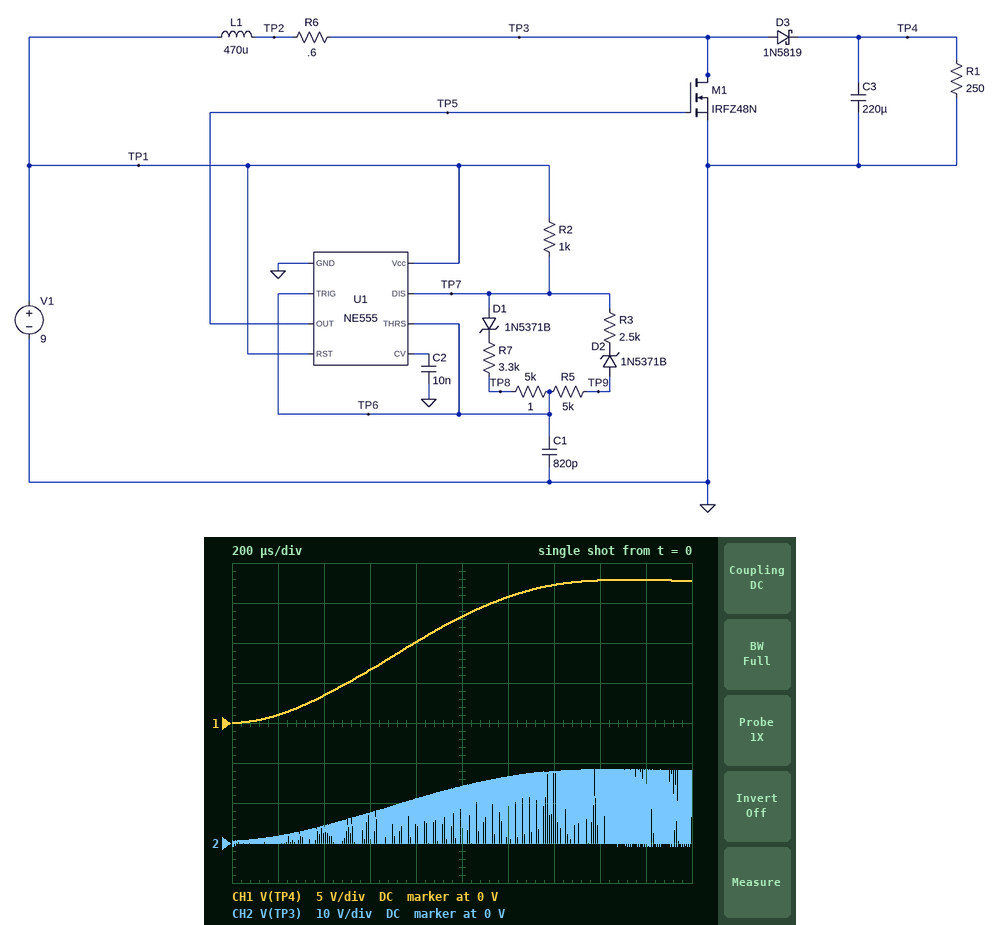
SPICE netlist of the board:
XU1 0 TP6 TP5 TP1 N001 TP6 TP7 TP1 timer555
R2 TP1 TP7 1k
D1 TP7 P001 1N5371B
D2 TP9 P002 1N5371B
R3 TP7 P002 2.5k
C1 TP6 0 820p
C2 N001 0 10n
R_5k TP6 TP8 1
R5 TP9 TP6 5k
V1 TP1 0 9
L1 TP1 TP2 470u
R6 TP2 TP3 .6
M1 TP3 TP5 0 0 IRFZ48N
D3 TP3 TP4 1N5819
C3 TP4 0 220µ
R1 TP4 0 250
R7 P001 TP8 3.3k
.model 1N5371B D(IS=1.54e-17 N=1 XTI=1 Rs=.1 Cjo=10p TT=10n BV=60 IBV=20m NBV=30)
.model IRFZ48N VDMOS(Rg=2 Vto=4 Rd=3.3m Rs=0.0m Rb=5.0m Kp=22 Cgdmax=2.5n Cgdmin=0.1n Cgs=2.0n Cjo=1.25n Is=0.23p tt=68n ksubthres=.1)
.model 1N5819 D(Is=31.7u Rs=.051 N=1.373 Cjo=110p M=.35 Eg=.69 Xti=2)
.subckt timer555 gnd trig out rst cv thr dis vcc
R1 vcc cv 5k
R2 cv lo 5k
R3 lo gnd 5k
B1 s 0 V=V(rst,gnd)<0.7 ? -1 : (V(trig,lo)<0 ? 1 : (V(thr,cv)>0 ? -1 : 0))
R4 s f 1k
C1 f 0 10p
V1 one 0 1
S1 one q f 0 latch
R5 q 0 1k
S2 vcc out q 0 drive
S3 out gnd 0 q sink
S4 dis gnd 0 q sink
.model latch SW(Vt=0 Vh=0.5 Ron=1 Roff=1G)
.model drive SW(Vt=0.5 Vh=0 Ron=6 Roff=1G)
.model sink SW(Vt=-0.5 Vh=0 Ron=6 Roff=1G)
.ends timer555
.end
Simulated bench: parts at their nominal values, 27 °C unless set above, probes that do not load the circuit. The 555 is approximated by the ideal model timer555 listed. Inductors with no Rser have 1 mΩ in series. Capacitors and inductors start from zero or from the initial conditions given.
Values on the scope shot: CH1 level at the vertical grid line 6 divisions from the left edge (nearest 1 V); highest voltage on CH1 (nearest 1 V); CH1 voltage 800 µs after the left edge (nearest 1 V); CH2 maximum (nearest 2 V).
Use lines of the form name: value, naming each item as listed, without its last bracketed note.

CH1 level at the vertical grid line 6 divisions from the left edge: 16 V
highest voltage on CH1: 18 V
CH1 voltage 800 µs after the left edge: 10 V
CH2 maximum: 18 V
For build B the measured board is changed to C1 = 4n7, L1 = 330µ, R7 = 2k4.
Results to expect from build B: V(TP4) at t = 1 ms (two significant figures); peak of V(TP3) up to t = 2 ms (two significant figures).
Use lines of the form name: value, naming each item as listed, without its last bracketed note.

V(TP4) at t = 1 ms: 15 V
peak of V(TP3) up to t = 2 ms: 16 V
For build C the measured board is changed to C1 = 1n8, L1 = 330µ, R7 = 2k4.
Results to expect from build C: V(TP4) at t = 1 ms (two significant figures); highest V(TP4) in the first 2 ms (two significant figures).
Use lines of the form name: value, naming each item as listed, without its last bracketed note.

V(TP4) at t = 1 ms: 15 V
highest V(TP4) in the first 2 ms: 16 V
